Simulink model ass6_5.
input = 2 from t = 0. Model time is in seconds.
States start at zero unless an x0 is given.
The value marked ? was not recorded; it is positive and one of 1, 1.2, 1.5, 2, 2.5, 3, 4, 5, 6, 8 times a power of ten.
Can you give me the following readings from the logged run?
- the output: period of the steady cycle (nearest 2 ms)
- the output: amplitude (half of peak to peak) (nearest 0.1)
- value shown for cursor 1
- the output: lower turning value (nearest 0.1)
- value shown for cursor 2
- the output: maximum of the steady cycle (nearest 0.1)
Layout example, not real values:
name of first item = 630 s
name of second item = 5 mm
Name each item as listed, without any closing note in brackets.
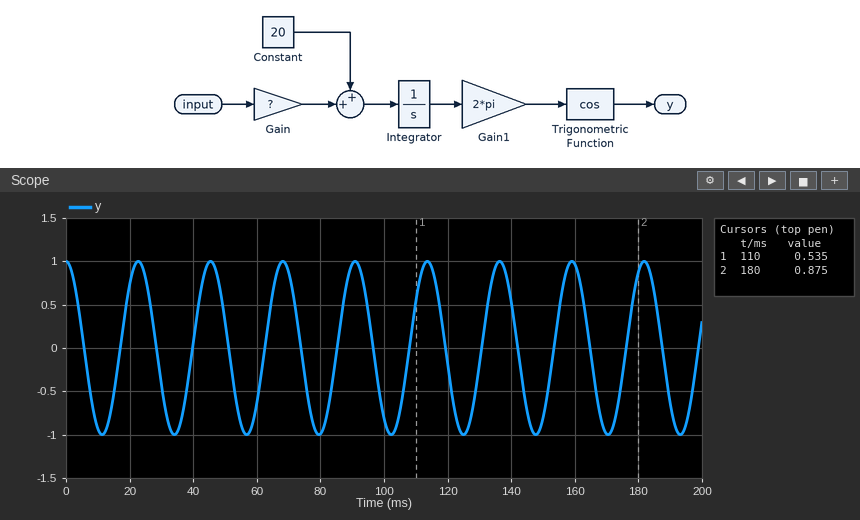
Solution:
the output: period of the steady cycle = 22 ms
the output: amplitude (half of peak to peak) = 1.0
value shown for cursor 1 = 0.535
the output: lower turning value = -1.0
value shown for cursor 2 = 0.875
the output: maximum of the steady cycle = 1.0
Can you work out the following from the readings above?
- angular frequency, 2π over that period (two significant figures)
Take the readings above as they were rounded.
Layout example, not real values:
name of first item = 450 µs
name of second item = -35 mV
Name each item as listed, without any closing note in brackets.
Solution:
angular frequency, 2π over that period = 0.29 rad/ms
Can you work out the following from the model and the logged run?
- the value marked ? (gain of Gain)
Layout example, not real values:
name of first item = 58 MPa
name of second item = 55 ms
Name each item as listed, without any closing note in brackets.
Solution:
the value marked ? = 12
